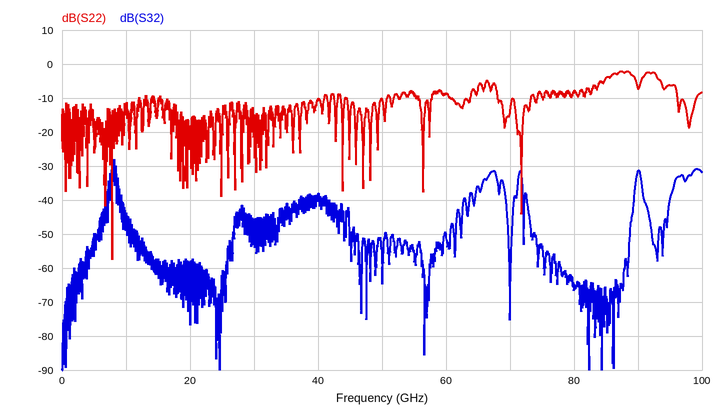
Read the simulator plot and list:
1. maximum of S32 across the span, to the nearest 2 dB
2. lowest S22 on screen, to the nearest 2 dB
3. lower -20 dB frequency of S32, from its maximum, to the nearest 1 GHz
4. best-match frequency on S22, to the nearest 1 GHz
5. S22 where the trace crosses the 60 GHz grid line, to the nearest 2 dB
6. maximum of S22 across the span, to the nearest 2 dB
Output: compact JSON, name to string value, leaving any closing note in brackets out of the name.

{"maximum of S32 across the span, to the nearest 2 dB": "-28 dB", "lowest S22 on screen, to the nearest 2 dB": "-58 dB", "lower -20 dB frequency of S32, from its maximum, to the nearest 1 GHz": "6 GHz", "best-match frequency on S22, to the nearest 1 GHz": "8 GHz", "S22 where the trace crosses the 60 GHz grid line, to the nearest 2 dB": "-8 dB", "maximum of S22 across the span, to the nearest 2 dB": "-2 dB"}
